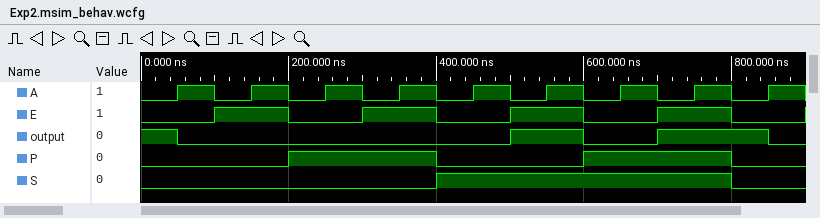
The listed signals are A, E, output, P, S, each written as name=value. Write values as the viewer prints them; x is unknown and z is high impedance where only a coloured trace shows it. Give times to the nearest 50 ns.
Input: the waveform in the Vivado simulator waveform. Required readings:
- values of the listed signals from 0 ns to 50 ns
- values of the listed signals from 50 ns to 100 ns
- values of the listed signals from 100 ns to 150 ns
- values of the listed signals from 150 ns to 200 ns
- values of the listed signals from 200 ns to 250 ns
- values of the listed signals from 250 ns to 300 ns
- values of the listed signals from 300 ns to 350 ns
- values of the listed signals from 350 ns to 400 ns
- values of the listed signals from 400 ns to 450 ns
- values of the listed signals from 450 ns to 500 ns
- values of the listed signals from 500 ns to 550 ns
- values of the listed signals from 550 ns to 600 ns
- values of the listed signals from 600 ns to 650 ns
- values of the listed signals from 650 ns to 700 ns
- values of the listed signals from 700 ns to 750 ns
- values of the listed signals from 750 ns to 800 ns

A=0, E=0, output=1, P=0, S=0
A=1, E=0, output=0, P=0, S=0
A=0, E=1, output=0, P=0, S=0
A=1, E=1, output=0, P=0, S=0
A=0, E=0, output=0, P=1, S=0
A=1, E=0, output=0, P=1, S=0
A=0, E=1, output=0, P=1, S=0
A=1, E=1, output=0, P=1, S=0
A=0, E=0, output=0, P=0, S=1
A=1, E=0, output=0, P=0, S=1
A=0, E=1, output=1, P=0, S=1
A=1, E=1, output=1, P=0, S=1
A=0, E=0, output=0, P=1, S=1
A=1, E=0, output=0, P=1, S=1
A=0, E=1, output=1, P=1, S=1
A=1, E=1, output=1, P=1, S=1
